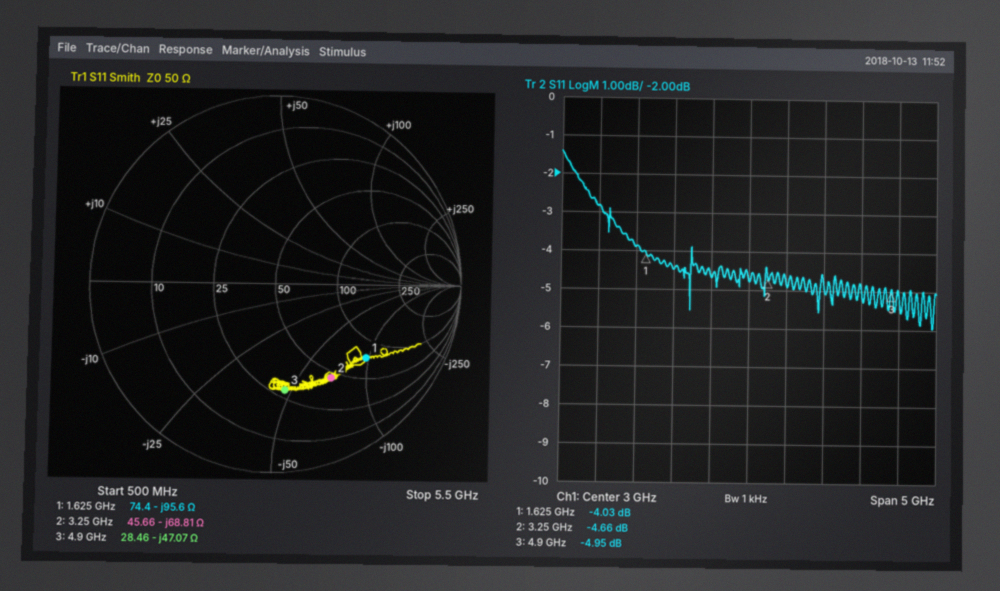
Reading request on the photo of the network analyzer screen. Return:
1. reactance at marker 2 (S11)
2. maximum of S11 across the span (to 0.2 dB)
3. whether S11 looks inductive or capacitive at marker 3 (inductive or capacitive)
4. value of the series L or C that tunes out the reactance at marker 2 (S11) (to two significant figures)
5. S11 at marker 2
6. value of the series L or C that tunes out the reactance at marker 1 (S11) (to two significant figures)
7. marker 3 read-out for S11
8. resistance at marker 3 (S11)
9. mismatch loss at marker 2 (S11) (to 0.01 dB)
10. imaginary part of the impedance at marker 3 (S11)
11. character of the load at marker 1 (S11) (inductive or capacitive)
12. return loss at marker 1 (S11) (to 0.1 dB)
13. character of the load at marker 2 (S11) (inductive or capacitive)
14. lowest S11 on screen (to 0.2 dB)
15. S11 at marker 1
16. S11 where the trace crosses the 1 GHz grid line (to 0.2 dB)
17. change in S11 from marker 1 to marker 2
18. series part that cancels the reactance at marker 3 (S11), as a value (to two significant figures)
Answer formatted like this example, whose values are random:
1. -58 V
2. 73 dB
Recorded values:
1. -68.81 Ω
2. -1.4 dB
3. capacitive
4. 3.4 nH
5. -4.66 dB
6. 9.4 nH
7. -4.95 dB
8. 28.46 Ω
9. 1.82 dB
10. -47.07 Ω
11. capacitive
12. 4.0 dB
13. capacitive
14. -6.0 dB
15. -4.03 dB
16. -2.8 dB
17. -0.63 dB
18. 1.5 nH
